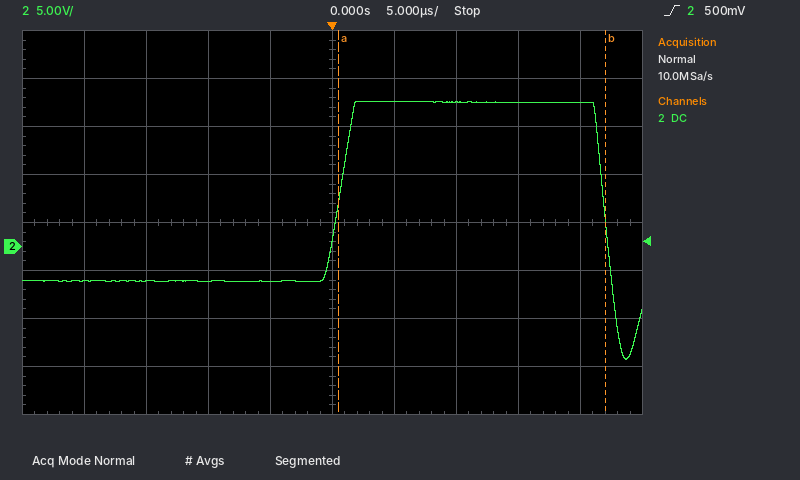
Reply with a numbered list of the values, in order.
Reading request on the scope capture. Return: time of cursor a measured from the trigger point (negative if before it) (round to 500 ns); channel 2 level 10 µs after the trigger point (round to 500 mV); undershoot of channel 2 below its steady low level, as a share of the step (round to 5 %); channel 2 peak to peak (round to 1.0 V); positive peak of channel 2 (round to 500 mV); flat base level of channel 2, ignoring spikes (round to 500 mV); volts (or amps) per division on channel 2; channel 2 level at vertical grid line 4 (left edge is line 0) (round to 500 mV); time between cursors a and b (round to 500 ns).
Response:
1. +500 ns
2. 15.0 V
3. 45 %
4. 27.0 V
5. 15.0 V
6. -3.5 V
7. 5 V
8. -3.5 V
9. 21.5 µs
